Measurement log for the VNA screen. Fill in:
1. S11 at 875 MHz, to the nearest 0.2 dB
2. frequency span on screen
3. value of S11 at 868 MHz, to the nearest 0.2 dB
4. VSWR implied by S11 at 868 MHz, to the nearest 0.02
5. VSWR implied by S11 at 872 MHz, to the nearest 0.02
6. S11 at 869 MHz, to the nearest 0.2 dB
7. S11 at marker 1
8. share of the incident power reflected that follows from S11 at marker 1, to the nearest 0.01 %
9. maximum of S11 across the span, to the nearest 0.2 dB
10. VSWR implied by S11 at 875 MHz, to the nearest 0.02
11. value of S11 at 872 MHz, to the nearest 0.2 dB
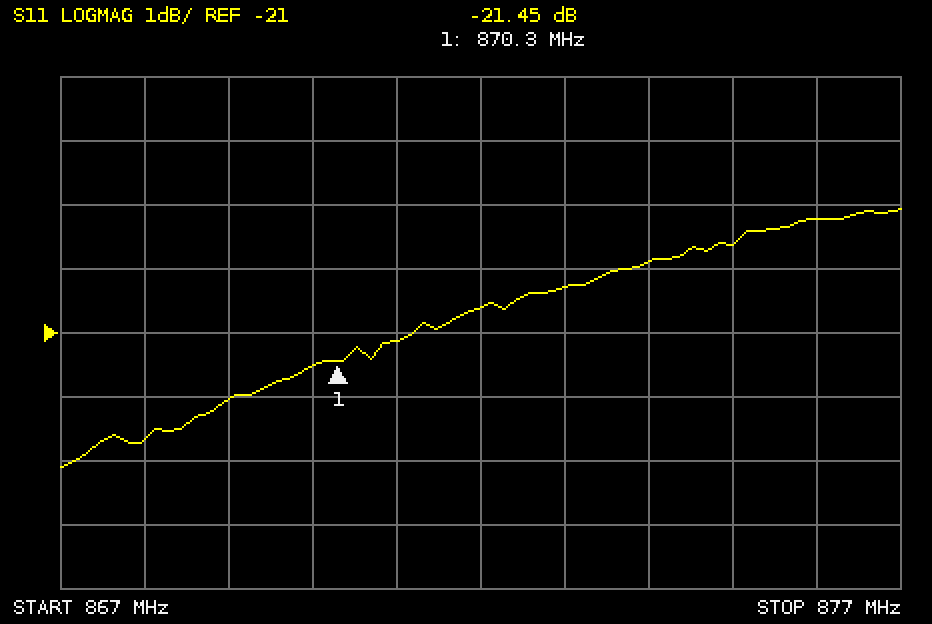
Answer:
-19.6 dB
10 MHz
-22.6 dB
1.16
1.20
-22.0 dB
-21.45 dB
0.72 %
-19.0 dB
1.24
-20.6 dB
